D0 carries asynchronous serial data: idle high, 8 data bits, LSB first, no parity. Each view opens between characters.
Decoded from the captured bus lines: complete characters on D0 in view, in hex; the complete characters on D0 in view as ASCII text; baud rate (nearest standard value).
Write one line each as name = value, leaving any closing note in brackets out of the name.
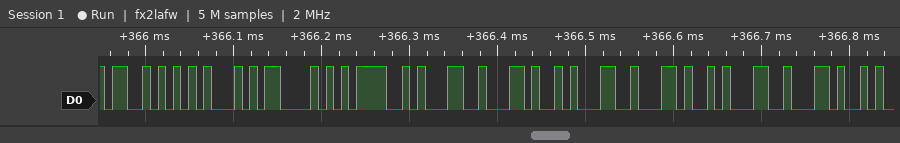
complete characters on D0 in view, in hex = 53, 45, 43, 3D, 31, 2C, 31, 2C, 31, 2C
the complete characters on D0 in view as ASCII text = "SEC=1,1,1,"
baud rate = 115200 baud
